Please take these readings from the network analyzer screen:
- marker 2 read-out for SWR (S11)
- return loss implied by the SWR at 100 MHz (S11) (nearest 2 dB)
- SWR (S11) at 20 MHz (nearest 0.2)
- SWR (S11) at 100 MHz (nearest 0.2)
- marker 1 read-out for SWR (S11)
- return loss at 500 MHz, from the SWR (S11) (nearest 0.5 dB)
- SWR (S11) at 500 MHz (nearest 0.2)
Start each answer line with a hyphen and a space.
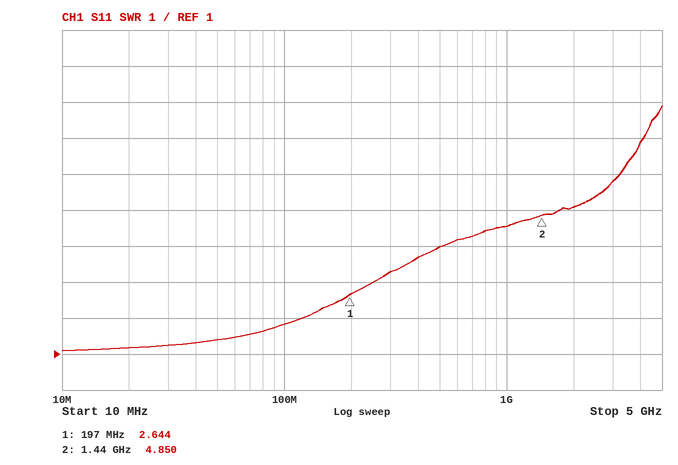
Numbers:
- 4.850
- 10 dB
- 1.2
- 1.8
- 2.644
- 4.5 dB
- 4.0
